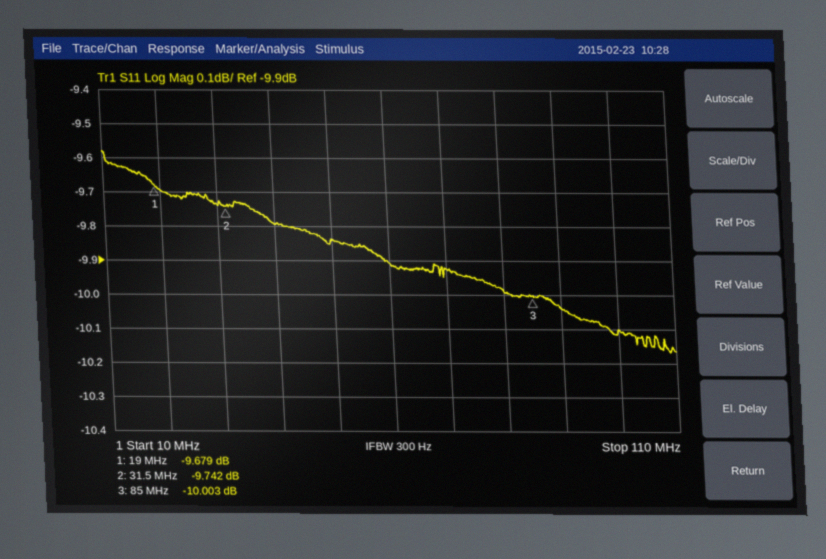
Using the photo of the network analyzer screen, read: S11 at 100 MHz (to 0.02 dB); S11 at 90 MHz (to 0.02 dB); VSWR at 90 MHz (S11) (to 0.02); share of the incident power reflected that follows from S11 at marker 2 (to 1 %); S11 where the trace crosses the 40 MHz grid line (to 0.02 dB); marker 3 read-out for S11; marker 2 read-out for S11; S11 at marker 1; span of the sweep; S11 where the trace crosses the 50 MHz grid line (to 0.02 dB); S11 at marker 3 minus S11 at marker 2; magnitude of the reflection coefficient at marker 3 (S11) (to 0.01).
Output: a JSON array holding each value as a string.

["-10.10 dB", "-10.04 dB", "1.92", "11 %", "-9.80 dB", "-10.003 dB", "-9.742 dB", "-9.679 dB", "100 MHz", "-9.84 dB", "-0.261 dB", "0.32"]
